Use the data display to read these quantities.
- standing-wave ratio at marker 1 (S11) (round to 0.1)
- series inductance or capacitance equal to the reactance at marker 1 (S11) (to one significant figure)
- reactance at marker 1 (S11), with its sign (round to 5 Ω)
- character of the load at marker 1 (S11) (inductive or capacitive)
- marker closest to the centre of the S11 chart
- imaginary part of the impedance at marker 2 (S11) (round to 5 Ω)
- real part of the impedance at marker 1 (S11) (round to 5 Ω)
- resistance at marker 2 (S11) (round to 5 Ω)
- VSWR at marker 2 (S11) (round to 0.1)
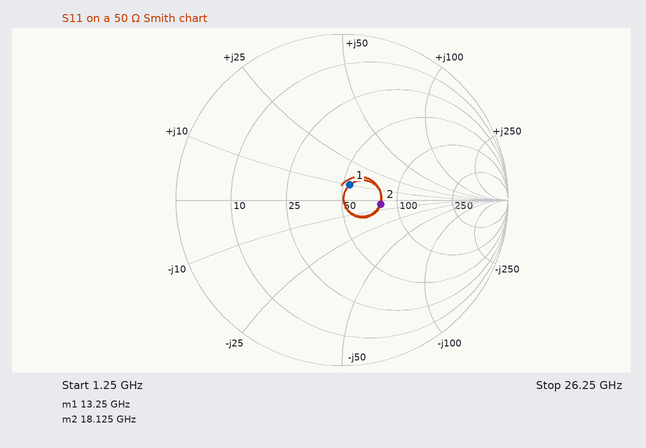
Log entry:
1.2
100 pH
+10 Ω
inductive
marker 1
-5 Ω
55 Ω
80 Ω
1.6
